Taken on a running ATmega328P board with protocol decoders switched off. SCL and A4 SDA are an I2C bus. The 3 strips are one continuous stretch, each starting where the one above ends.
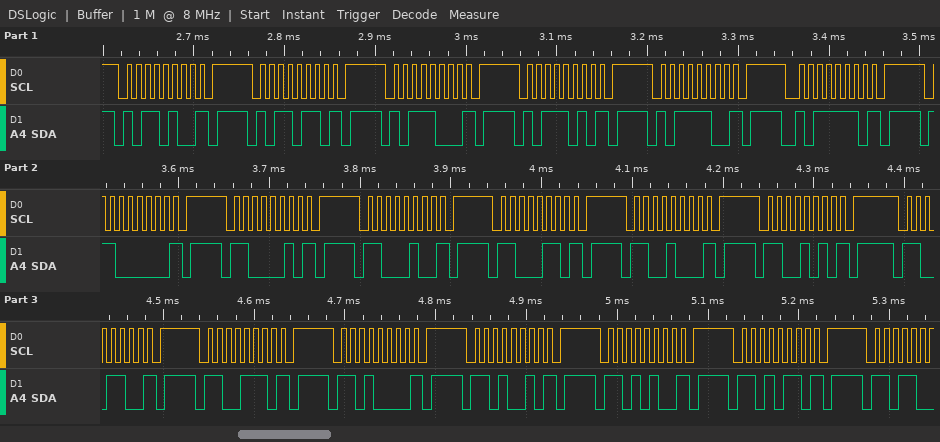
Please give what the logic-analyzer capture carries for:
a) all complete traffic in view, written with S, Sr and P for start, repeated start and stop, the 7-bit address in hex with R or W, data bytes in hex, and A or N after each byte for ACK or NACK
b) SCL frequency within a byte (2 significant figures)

S 5AW N P S 5BW N P S 5CW N P S 5DW N P S 5EW N P S 5FW N P S 60W N P S 61W N P S 62W N P S 63W N P S 64W N P S 65W N P S 66W N P S 67W N P S 68W N P S 69W N P S 6AW N P S 6BW N P
100 kHz
